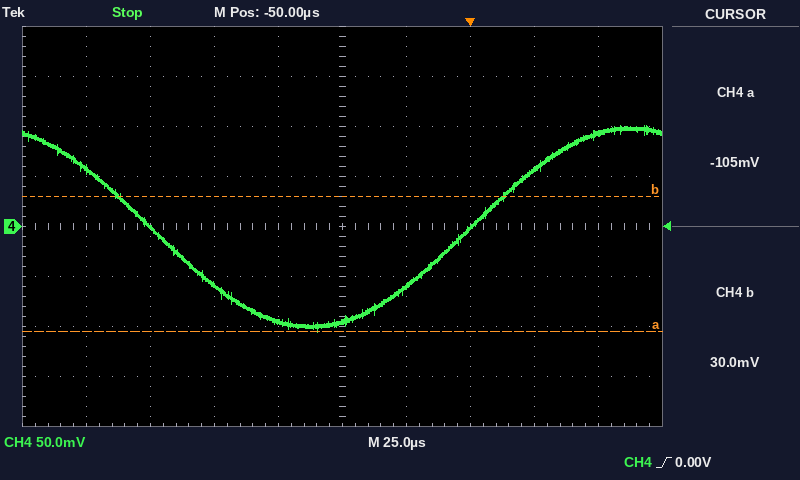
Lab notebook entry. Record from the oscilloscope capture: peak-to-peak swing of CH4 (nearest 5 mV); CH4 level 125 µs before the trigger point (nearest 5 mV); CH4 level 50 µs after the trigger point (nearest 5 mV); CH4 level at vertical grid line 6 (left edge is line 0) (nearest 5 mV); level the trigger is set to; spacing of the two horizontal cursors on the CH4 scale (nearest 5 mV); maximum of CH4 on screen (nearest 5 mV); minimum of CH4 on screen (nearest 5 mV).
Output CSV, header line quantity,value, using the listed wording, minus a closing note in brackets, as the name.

quantity,value
peak-to-peak swing of CH4,205 mV
CH4 level 125 µs before the trigger point,0 mV
CH4 level 50 µs after the trigger point,95 mV
CH4 level at vertical grid line 6 (left edge is line 0),-60 mV
level the trigger is set to,0.00 V
spacing of the two horizontal cursors on the CH4 scale,135 mV
maximum of CH4 on screen,100 mV
minimum of CH4 on screen,-105 mV
